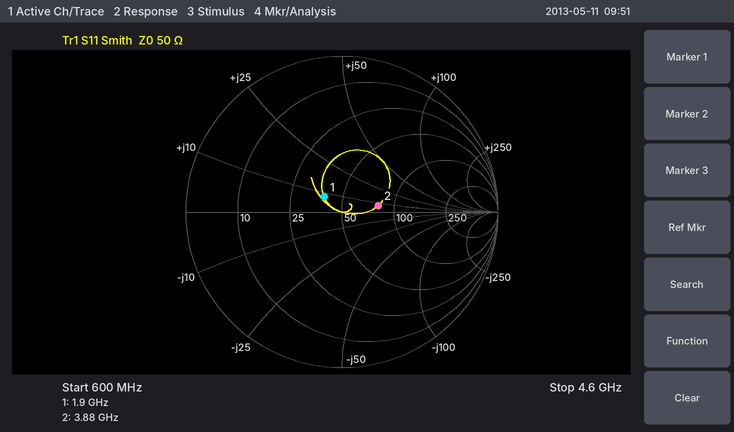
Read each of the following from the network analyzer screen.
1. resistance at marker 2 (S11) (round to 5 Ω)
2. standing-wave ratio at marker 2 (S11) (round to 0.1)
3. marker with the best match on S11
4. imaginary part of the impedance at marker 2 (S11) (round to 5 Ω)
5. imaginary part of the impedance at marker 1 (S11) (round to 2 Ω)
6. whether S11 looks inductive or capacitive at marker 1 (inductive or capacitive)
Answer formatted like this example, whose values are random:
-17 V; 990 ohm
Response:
80 Ω; 1.6; marker 1; +5 Ω; +8 Ω; inductive
